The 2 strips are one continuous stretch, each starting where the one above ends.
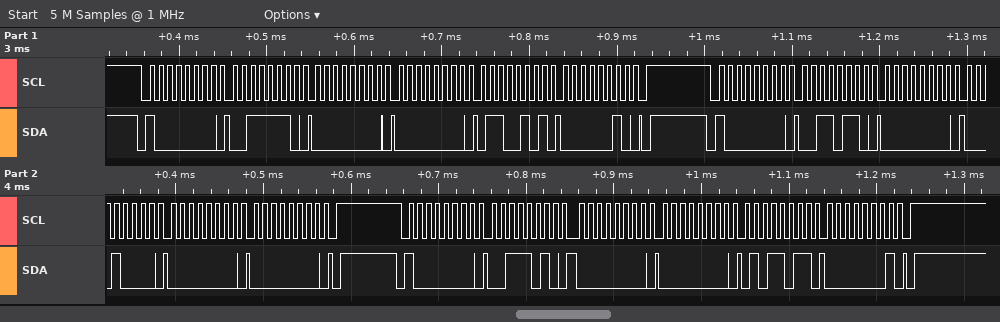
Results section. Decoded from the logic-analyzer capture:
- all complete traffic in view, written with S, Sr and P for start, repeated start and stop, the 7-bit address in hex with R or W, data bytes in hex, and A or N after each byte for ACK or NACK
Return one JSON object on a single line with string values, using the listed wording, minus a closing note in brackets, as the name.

{"all complete traffic in view, written with S, Sr and P for start, repeated start and stop, the 7-bit address in hex with R or W, data bytes in hex, and A or N after each byte for ACK or NACK": "S 40W A 3E A 00 A 00 A 65 A 02 A P S 40W A 36 A 00 A 10 A 00 A 00 A P S 40W A 3A A 00 A 00 A 5B A 01 A P"}
